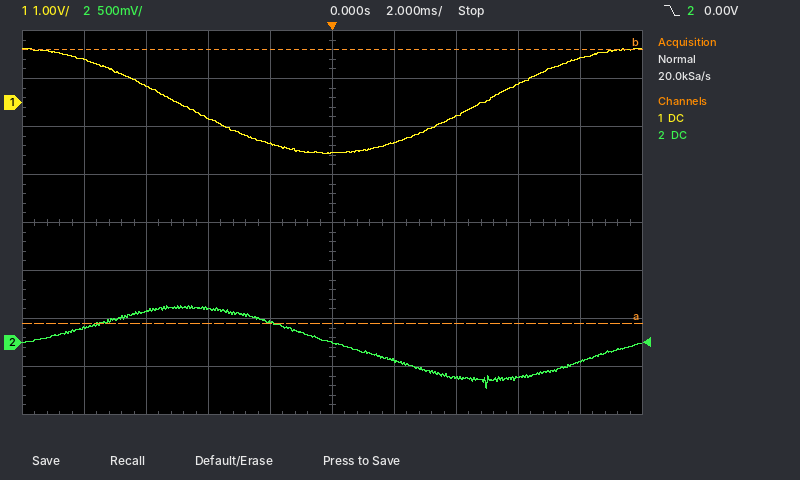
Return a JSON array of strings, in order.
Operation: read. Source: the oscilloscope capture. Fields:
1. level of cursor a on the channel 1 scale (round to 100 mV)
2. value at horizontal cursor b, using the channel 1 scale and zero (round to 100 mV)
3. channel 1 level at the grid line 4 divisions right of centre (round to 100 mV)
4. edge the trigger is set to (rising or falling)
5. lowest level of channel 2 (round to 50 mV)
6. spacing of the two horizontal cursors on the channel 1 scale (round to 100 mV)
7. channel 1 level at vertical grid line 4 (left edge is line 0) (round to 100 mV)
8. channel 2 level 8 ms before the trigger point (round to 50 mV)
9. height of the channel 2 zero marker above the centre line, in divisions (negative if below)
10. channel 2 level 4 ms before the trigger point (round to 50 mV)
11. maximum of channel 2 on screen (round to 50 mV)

["-4.6 V", "1.1 V", "900 mV", "falling", "-500 mV", "5.7 V", "-900 mV", "150 mV", "-2.5 div", "350 mV", "400 mV"]
